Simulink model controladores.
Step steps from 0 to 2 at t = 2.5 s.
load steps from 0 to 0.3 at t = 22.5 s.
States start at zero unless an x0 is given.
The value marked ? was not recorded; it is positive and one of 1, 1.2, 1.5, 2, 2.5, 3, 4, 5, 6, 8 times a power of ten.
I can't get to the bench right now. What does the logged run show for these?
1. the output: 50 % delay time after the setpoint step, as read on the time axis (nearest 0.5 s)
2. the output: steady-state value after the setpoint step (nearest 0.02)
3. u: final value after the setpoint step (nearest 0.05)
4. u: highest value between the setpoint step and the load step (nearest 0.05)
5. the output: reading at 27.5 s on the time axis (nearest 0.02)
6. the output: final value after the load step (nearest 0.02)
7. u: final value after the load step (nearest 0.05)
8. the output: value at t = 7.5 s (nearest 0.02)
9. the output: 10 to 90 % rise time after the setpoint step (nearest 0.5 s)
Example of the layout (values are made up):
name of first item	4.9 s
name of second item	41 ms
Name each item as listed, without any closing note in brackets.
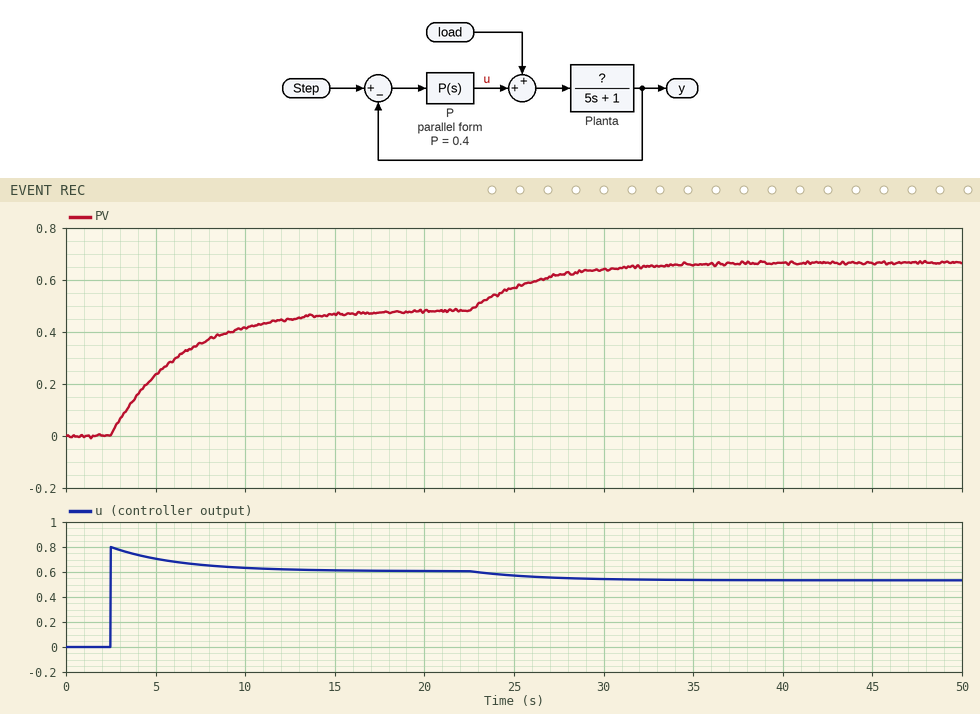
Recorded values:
the output: 50 % delay time after the setpoint step, as read on the time axis	5.0 s
the output: steady-state value after the setpoint step	0.48
u: final value after the setpoint step	0.60
u: highest value between the setpoint step and the load step	0.80
the output: reading at 27.5 s on the time axis	0.62
the output: final value after the load step	0.66
u: final value after the load step	0.55
the output: value at t = 7.5 s	0.36
the output: 10 to 90 % rise time after the setpoint step	8.5 s
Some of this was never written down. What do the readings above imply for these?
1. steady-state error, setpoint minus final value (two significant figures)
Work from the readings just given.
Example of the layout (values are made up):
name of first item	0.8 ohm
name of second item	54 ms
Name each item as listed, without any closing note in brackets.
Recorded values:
steady-state error, setpoint minus final value	1.5
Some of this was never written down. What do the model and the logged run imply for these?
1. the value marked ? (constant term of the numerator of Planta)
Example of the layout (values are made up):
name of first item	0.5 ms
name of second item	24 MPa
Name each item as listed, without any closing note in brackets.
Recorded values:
the value marked ?	0.8
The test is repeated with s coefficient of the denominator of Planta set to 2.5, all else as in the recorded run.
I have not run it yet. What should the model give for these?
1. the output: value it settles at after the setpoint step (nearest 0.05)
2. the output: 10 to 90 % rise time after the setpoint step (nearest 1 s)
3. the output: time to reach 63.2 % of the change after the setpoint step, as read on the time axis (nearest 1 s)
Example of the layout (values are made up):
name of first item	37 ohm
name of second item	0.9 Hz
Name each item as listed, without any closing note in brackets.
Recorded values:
the output: value it settles at after the setpoint step	0.50
the output: 10 to 90 % rise time after the setpoint step	4 s
the output: time to reach 63.2 % of the change after the setpoint step, as read on the time axis	4 s
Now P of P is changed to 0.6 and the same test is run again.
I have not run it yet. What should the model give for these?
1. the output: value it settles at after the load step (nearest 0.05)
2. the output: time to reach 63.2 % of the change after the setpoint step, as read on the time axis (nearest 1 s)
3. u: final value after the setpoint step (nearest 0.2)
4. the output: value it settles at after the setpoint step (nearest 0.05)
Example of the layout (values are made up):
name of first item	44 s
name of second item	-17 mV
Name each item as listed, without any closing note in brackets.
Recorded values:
the output: value it settles at after the load step	0.80
the output: time to reach 63.2 % of the change after the setpoint step, as read on the time axis	6 s
u: final value after the setpoint step	0.8
the output: value it settles at after the setpoint step	0.65
